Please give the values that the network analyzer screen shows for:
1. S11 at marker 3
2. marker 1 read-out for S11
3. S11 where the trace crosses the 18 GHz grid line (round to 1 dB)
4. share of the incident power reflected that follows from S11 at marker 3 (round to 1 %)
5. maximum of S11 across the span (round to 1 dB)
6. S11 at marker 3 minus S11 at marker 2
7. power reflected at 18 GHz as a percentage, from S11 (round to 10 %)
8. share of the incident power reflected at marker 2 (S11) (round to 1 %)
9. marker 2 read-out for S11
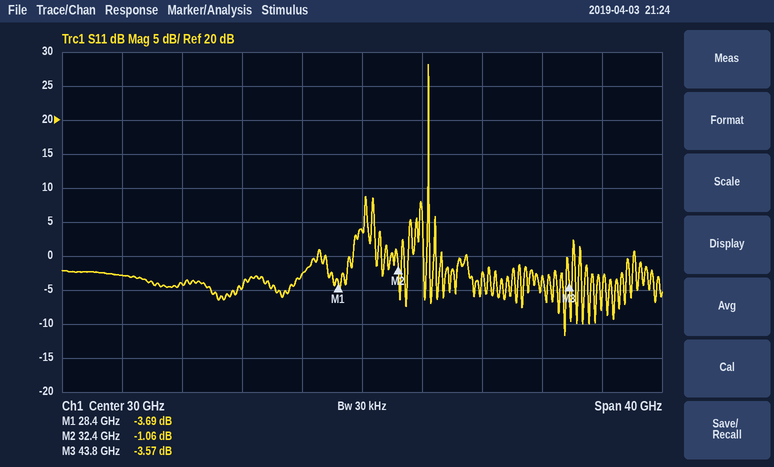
-3.57 dB
-3.69 dB
-4 dB
44 %
28 dB
-2.51 dB
40 %
78 %
-1.06 dB
